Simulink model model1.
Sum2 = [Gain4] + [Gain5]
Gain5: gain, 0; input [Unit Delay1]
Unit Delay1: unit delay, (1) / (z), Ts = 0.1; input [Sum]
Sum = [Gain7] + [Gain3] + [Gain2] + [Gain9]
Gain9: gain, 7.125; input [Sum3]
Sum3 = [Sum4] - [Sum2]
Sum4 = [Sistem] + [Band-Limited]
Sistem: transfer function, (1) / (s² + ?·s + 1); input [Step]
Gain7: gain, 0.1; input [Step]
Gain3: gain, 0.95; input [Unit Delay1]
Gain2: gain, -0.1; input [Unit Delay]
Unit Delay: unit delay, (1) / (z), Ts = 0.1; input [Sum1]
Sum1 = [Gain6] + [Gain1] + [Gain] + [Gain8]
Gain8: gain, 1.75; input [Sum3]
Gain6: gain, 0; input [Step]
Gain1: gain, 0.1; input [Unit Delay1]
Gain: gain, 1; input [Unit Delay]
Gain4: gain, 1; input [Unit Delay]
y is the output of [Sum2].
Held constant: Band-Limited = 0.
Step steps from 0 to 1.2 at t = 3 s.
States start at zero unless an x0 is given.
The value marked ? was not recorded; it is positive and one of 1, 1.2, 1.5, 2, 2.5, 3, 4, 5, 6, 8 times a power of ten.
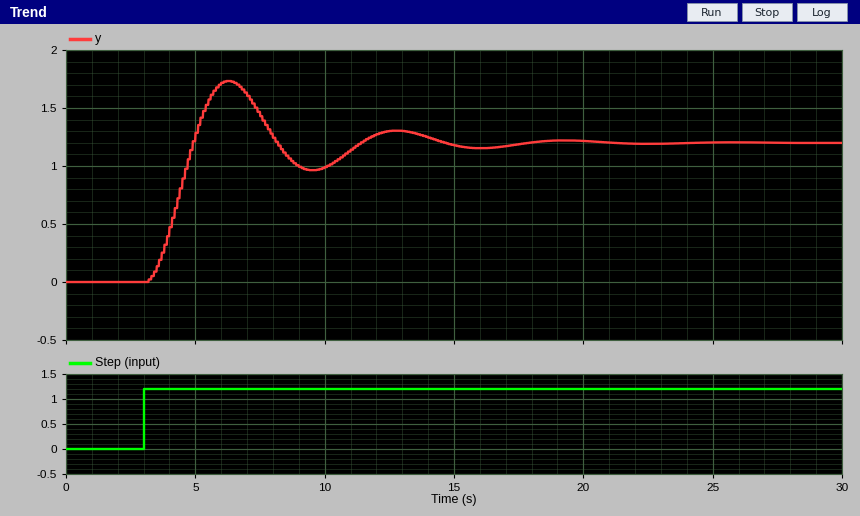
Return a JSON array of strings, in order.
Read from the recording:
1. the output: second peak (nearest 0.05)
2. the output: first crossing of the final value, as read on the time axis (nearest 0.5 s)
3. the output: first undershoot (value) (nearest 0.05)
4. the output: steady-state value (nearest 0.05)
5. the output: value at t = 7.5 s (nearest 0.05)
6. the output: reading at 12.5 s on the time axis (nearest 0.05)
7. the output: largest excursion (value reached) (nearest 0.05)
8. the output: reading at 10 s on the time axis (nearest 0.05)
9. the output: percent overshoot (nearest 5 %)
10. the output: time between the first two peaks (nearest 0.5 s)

["1.30", "5.0 s", "0.95", "1.20", "1.45", "1.30", "1.75", "1.00", "45 %", "6.5 s"]
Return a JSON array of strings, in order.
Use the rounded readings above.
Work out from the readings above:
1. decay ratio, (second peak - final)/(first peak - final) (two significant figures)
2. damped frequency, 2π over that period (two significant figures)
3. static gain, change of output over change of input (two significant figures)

["0.18", "0.97 rad/s", "1.0"]
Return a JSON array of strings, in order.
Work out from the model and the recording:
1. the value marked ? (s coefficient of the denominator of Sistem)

["0.5"]
